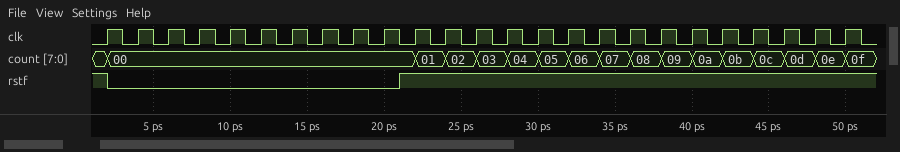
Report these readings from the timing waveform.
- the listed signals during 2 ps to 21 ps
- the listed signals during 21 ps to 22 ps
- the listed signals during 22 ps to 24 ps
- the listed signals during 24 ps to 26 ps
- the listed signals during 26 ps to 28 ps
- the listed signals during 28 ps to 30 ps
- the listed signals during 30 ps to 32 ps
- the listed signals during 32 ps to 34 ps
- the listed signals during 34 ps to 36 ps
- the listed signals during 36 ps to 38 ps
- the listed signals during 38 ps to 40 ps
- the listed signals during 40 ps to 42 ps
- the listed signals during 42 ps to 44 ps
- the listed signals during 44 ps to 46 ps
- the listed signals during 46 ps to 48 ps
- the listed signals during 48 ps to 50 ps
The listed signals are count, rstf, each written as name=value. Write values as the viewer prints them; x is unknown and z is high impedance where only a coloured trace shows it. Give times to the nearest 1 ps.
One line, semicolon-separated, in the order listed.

count=00, rstf=0; count=00, rstf=1; count=01, rstf=1; count=02, rstf=1; count=03, rstf=1; count=04, rstf=1; count=05, rstf=1; count=06, rstf=1; count=07, rstf=1; count=08, rstf=1; count=09, rstf=1; count=0a, rstf=1; count=0b, rstf=1; count=0c, rstf=1; count=0d, rstf=1; count=0e, rstf=1
